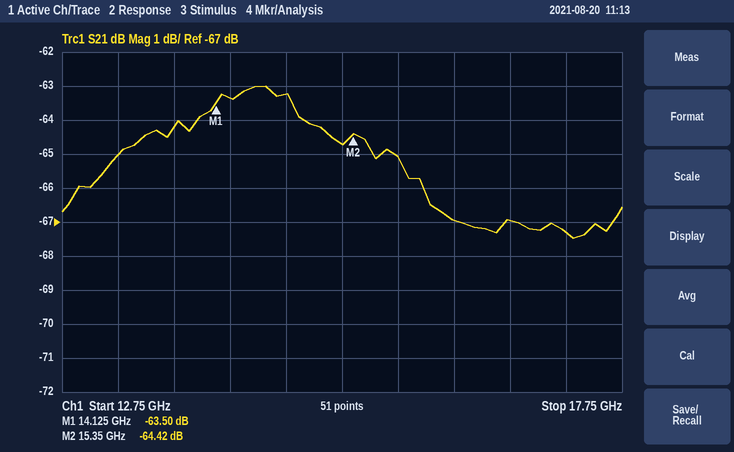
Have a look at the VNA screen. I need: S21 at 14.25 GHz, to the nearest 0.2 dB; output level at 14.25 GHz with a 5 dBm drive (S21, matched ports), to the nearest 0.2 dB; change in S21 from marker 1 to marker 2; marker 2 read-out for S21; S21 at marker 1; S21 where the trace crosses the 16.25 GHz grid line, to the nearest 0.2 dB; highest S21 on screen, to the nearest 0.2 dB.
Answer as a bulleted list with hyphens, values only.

- -63.4 dB
- -58.4 dBm
- -0.92 dB
- -64.42 dB
- -63.50 dB
- -67.0 dB
- -63.0 dB
